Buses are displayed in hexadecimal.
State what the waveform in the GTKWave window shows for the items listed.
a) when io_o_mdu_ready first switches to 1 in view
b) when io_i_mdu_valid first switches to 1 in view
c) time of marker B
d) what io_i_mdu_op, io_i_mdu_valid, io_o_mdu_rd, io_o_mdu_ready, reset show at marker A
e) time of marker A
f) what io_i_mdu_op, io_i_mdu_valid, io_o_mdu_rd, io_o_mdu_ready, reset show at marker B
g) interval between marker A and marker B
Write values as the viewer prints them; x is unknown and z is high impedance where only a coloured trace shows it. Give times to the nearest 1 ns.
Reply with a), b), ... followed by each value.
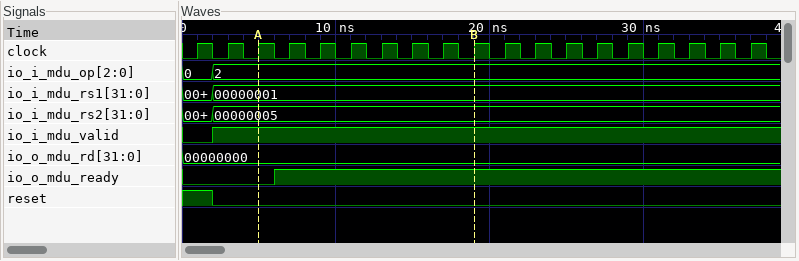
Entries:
a) 6 ns
b) 2 ns
c) 19 ns
d) io_i_mdu_op=2, io_i_mdu_valid=1, io_o_mdu_rd=00000000, io_o_mdu_ready=0, reset=0
e) 5 ns
f) io_i_mdu_op=2, io_i_mdu_valid=1, io_o_mdu_rd=00000000, io_o_mdu_ready=1, reset=0
g) 14 ns
